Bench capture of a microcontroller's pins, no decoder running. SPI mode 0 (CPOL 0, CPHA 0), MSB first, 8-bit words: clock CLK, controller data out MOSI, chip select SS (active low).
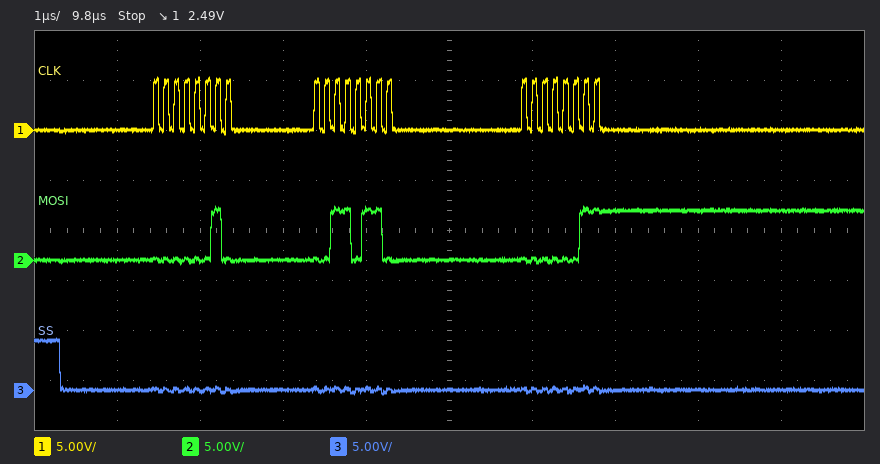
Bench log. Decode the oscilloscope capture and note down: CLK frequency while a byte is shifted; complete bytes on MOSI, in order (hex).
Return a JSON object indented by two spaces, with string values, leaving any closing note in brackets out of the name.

{
  "CLK frequency while a byte is shifted": "8 MHz",
  "complete bytes on MOSI, in order": "02 36 03"
}
